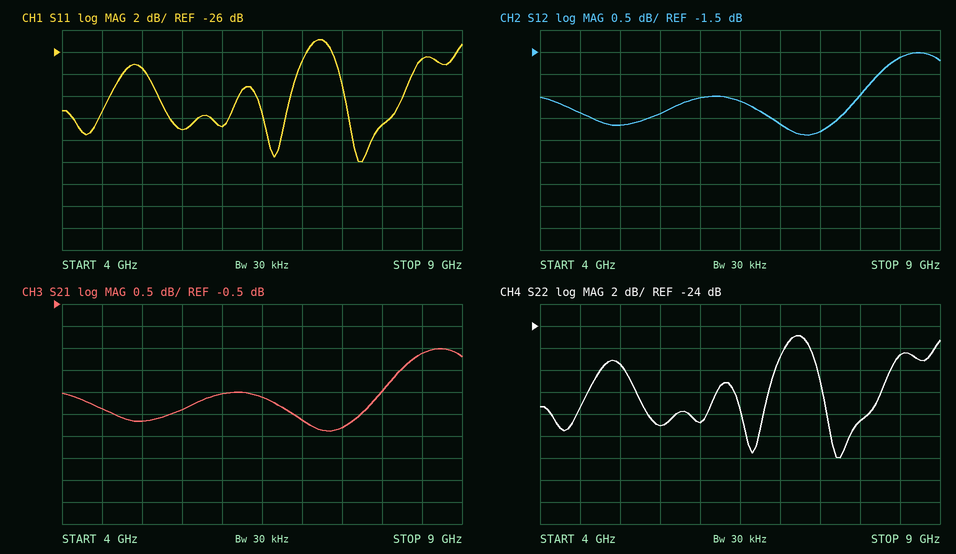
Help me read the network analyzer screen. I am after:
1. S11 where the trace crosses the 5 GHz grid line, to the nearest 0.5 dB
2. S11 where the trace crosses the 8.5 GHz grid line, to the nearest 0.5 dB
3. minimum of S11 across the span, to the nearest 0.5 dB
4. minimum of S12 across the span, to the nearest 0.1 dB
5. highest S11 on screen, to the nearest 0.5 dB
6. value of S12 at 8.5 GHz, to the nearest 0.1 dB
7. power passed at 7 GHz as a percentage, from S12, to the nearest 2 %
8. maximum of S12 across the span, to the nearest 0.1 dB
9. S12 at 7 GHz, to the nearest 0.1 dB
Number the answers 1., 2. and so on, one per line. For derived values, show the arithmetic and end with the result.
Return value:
1. -27.5 dB
2. -26.5 dB
3. -36.0 dB
4. -3.4 dB
5. -25.0 dB
6. -1.6 dB
7. 10^(-3.1/10) ≈ 49.0 %, so 48 % to the nearest 2 %
8. -1.5 dB
9. -3.1 dB
